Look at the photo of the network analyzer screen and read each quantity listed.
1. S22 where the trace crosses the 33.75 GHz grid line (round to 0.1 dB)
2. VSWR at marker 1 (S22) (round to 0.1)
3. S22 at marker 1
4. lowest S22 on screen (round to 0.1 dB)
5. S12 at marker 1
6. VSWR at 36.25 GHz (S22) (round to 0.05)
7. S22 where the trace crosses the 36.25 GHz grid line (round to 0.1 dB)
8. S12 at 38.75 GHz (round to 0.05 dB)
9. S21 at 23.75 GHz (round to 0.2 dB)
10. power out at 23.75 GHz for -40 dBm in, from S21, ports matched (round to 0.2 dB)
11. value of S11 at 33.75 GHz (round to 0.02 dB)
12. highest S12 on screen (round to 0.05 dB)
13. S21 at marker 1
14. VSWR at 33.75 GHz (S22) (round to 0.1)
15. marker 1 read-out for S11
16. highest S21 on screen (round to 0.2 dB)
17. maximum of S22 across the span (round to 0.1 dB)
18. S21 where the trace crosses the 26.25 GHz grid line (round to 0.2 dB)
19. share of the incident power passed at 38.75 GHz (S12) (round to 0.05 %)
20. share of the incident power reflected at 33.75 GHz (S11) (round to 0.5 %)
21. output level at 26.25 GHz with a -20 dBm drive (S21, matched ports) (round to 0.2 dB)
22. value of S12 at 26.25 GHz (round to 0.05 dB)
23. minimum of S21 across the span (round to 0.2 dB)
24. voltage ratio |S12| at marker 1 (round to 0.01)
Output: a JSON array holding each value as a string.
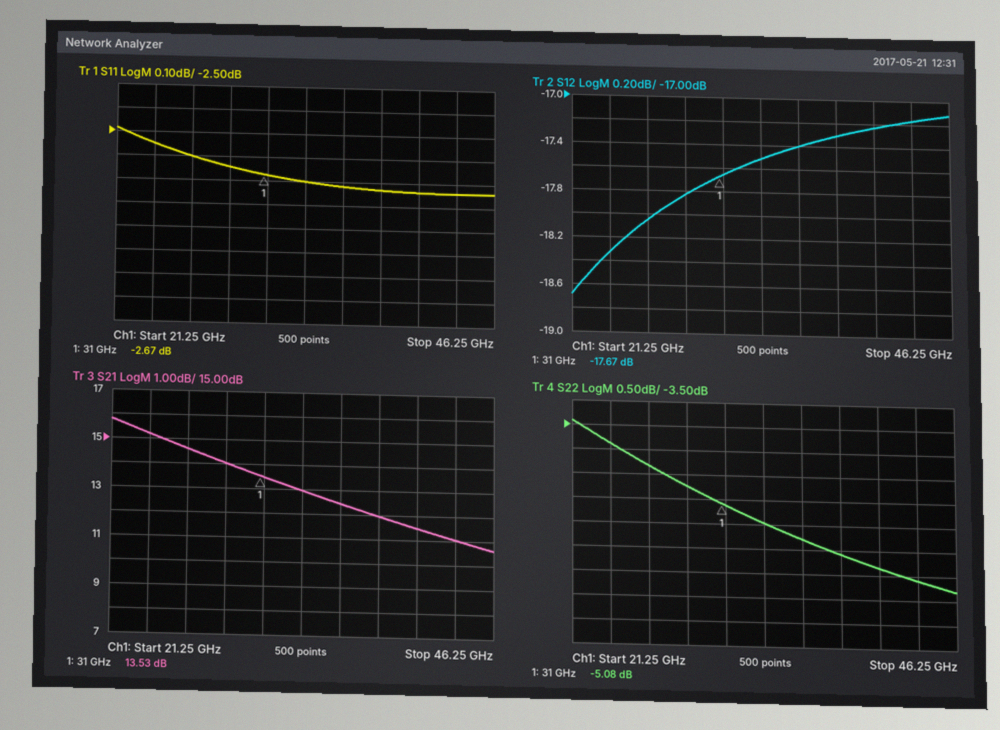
["-5.5 dB", "3.5", "-5.08 dB", "-6.8 dB", "-17.67 dB", "3.10", "-5.8 dB", "-17.30 dB", "15.2 dB", "-24.8 dBm", "-2.70 dB", "-17.10 dB", "13.53 dB", "3.3", "-2.67 dB", "15.8 dB", "-3.4 dB", "14.6 dB", "1.85 %", "53.5 %", "-5.4 dBm", "-18.05 dB", "10.6 dB", "0.13"]
